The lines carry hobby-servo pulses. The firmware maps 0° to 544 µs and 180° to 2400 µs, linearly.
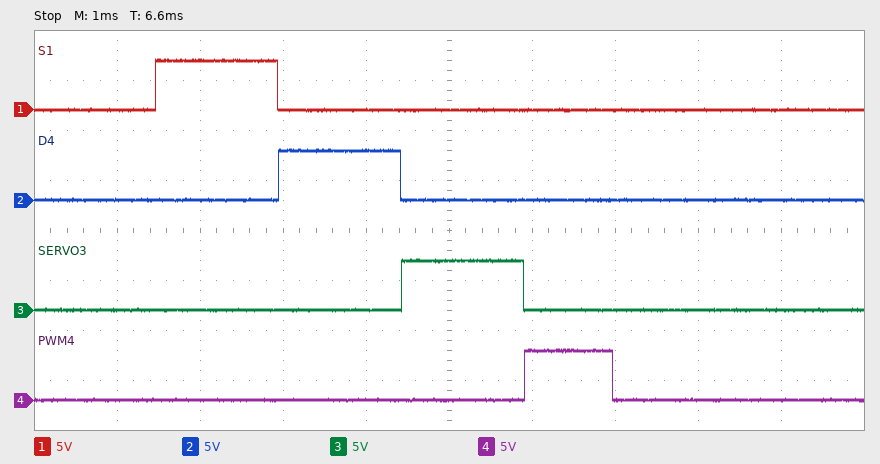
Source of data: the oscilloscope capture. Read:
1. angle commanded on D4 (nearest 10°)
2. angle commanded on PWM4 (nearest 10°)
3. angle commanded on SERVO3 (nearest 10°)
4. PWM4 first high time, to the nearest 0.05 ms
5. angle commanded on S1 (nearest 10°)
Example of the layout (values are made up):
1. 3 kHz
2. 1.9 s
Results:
1. 90°
2. 50°
3. 90°
4. 1.05 ms
5. 90°
